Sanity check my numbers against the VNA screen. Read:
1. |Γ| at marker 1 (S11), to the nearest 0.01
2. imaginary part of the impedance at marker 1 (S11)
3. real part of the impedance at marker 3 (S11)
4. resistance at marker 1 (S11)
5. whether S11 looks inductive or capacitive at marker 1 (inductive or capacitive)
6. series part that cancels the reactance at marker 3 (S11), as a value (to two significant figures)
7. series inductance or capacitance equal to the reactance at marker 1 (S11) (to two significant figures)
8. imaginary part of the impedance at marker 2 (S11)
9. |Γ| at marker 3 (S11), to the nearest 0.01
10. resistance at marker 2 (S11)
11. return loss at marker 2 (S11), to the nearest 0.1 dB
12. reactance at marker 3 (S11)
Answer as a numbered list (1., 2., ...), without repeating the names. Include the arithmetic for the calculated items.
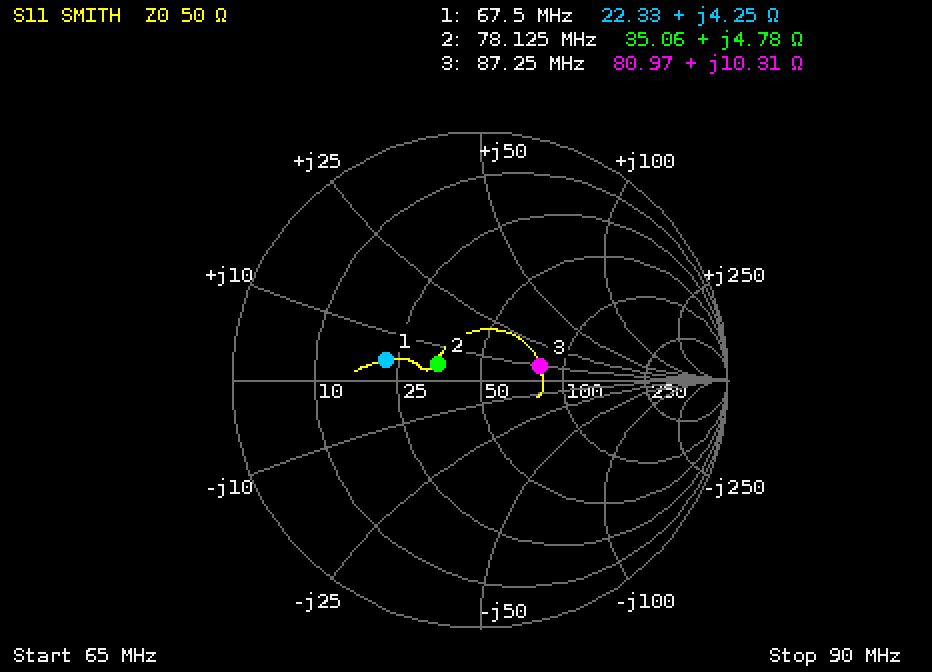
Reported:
1. 0.39
2. +4.25 Ω
3. 80.97 Ω
4. 22.33 Ω
5. inductive
6. C = 1/(2π × 87.25 MHz × 10.31 Ω) ≈ 177 pF, so 180 pF to two significant figures
7. L = 4.25 Ω/(2π × 67.5 MHz) ≈ 10 nH
8. +4.78 Ω
9. 0.25
10. 35.06 Ω
11. 14.7 dB
12. +10.31 Ω
